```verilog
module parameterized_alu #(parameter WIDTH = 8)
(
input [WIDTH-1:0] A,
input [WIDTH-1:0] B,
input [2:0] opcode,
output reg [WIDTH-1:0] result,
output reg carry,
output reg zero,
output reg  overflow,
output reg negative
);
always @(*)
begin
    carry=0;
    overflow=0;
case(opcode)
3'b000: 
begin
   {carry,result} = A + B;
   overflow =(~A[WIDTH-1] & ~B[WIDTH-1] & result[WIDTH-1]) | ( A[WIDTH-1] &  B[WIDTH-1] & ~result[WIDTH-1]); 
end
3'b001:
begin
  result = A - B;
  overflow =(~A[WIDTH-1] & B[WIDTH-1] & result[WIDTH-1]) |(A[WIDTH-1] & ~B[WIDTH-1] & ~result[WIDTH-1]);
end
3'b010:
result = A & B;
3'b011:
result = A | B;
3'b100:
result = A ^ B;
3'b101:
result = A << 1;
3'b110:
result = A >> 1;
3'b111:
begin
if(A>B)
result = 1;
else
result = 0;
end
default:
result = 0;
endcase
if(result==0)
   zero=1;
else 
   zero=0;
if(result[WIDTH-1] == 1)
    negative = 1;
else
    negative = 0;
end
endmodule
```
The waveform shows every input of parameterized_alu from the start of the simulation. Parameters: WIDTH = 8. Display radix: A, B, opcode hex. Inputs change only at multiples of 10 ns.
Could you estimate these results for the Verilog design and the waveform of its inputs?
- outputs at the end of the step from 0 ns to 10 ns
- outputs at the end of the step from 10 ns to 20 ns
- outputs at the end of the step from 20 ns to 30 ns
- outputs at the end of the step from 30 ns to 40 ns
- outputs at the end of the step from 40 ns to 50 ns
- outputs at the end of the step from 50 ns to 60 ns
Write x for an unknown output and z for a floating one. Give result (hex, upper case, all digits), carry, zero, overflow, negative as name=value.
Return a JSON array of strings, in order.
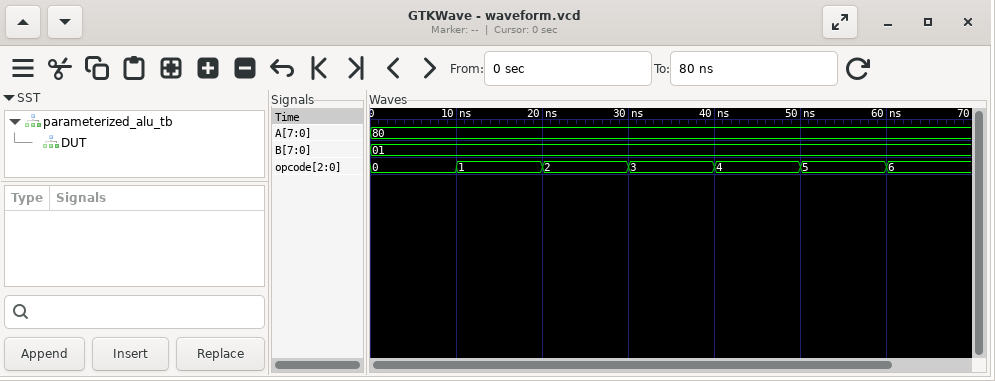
["result=81, carry=0, zero=0, overflow=0, negative=1", "result=7F, carry=0, zero=0, overflow=1, negative=0", "result=00, carry=0, zero=1, overflow=0, negative=0", "result=81, carry=0, zero=0, overflow=0, negative=1", "result=81, carry=0, zero=0, overflow=0, negative=1", "result=00, carry=0, zero=1, overflow=0, negative=0"]
